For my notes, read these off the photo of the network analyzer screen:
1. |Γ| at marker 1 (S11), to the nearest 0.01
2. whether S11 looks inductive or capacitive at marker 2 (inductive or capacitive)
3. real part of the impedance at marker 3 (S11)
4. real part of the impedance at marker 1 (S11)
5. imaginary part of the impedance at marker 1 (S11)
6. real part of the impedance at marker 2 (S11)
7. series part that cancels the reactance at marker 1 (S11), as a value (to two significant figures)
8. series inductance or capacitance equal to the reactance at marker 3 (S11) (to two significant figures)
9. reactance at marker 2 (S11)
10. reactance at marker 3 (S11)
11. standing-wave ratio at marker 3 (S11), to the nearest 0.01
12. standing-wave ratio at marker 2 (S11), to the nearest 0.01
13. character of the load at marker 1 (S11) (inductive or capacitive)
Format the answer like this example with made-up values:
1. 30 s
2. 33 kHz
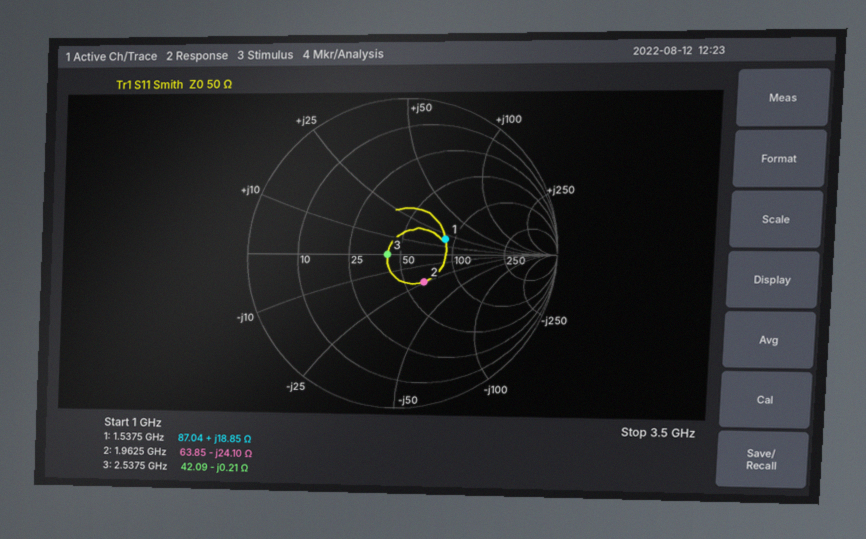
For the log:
1. 0.30
2. capacitive
3. 42.09 Ω
4. 87.04 Ω
5. +18.85 Ω
6. 63.85 Ω
7. 5.5 pF
8. 300 pF
9. -24.10 Ω
10. -0.21 Ω
11. 1.19
12. 1.63
13. inductive
